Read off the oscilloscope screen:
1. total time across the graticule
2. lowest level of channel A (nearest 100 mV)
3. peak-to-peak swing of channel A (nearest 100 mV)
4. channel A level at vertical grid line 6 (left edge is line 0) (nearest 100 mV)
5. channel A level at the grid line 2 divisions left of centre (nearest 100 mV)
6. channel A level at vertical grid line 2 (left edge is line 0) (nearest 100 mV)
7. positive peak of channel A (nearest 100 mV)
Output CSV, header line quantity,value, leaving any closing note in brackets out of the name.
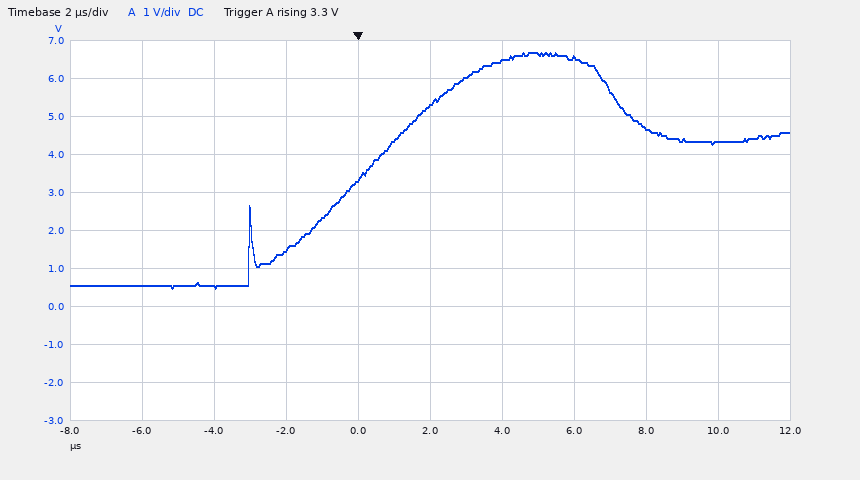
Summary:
quantity,value
total time across the graticule,20 µs
lowest level of channel A,500 mV
peak-to-peak swing of channel A,6.2 V
channel A level at vertical grid line 6 (left edge is line 0),6.5 V
channel A level at the grid line 2 divisions left of centre,1.5 V
channel A level at vertical grid line 2 (left edge is line 0),500 mV
positive peak of channel A,6.7 V
